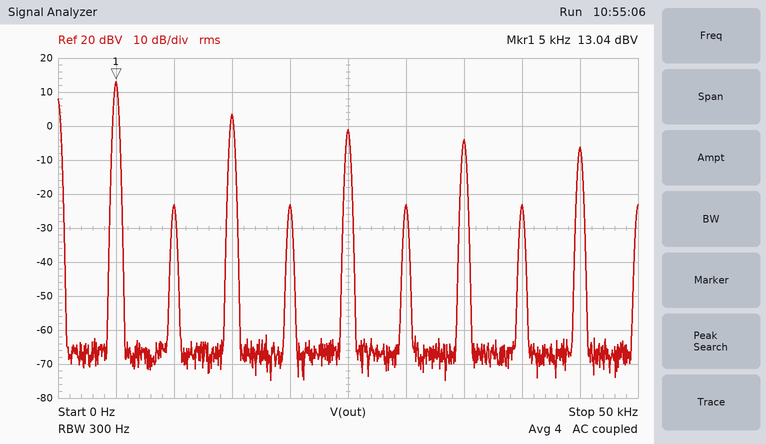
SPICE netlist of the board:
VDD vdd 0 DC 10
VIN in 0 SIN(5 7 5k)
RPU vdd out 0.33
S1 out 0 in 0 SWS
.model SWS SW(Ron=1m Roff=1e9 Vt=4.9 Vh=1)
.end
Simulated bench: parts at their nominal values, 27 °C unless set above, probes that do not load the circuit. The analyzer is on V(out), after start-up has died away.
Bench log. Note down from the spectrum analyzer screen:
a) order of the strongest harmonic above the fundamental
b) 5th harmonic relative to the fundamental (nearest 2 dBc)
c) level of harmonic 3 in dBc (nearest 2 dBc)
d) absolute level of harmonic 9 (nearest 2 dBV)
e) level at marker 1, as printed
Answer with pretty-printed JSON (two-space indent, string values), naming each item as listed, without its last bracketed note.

{
  "order of the strongest harmonic above the fundamental": "3",
  "5th harmonic relative to the fundamental": "-14 dBc",
  "level of harmonic 3 in dBc": "-10 dBc",
  "absolute level of harmonic 9": "-6 dBV",
  "level at marker 1, as printed": "13.04 dBV"
}
